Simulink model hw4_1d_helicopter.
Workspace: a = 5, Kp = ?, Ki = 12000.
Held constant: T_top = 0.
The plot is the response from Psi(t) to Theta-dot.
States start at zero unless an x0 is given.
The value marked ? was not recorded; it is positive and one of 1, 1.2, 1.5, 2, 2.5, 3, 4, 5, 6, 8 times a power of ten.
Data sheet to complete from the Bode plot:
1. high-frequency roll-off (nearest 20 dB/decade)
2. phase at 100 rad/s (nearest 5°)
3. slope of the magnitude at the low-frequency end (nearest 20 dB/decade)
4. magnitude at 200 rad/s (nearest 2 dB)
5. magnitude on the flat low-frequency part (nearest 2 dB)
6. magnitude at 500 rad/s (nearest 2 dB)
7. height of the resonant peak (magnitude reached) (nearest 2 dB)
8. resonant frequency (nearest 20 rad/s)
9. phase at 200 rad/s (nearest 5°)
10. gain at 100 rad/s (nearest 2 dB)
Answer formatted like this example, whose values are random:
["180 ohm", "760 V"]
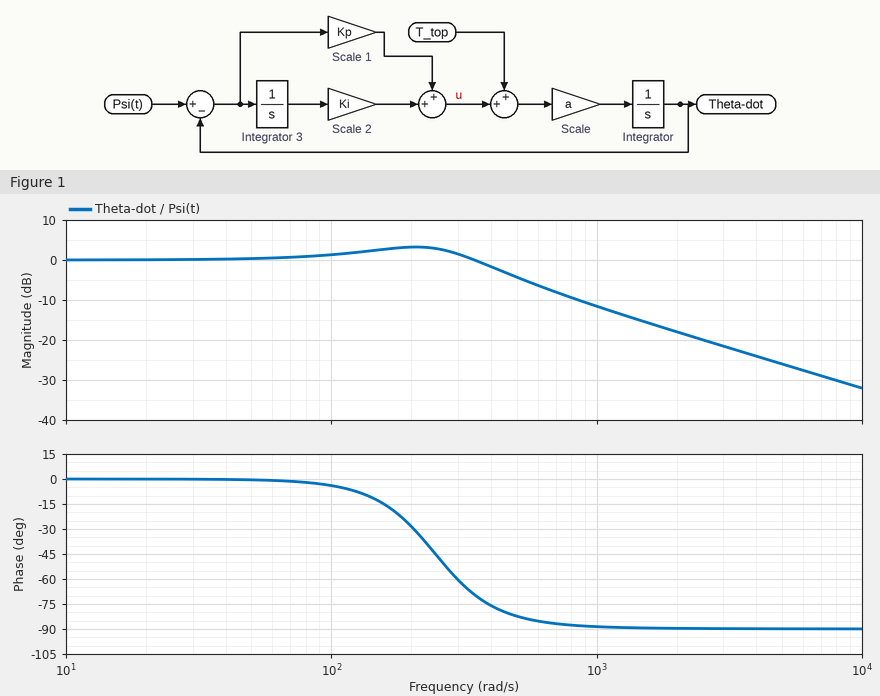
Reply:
["-20 dB/decade", "-5°", "0 dB/decade", "4 dB", "0 dB", "-4 dB", "4 dB", "200 rad/s", "-30°", "2 dB"]
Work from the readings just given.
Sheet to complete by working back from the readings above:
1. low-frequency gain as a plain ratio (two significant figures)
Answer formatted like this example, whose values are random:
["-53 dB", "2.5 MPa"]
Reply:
["1.0"]
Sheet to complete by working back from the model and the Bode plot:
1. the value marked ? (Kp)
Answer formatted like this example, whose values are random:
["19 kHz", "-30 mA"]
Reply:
["50"]
